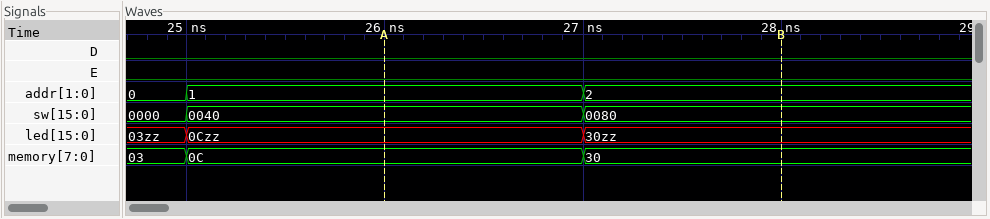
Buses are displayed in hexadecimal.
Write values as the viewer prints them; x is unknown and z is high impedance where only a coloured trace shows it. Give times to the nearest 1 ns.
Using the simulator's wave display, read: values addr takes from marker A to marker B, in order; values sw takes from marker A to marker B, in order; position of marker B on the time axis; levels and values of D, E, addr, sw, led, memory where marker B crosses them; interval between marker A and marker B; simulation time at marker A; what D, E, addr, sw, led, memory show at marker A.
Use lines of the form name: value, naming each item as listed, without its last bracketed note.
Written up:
values addr takes from marker A to marker B, in order: 1, 2
values sw takes from marker A to marker B, in order: 0040, 0080
position of marker B on the time axis: 28 ns
levels and values of D, E, addr, sw, led, memory where marker B crosses them: D=0, E=0, addr=2, sw=0080, led=30zz, memory=30
interval between marker A and marker B: 2 ns
simulation time at marker A: 26 ns
what D, E, addr, sw, led, memory show at marker A: D=0, E=0, addr=1, sw=0040, led=0Czz, memory=0C
